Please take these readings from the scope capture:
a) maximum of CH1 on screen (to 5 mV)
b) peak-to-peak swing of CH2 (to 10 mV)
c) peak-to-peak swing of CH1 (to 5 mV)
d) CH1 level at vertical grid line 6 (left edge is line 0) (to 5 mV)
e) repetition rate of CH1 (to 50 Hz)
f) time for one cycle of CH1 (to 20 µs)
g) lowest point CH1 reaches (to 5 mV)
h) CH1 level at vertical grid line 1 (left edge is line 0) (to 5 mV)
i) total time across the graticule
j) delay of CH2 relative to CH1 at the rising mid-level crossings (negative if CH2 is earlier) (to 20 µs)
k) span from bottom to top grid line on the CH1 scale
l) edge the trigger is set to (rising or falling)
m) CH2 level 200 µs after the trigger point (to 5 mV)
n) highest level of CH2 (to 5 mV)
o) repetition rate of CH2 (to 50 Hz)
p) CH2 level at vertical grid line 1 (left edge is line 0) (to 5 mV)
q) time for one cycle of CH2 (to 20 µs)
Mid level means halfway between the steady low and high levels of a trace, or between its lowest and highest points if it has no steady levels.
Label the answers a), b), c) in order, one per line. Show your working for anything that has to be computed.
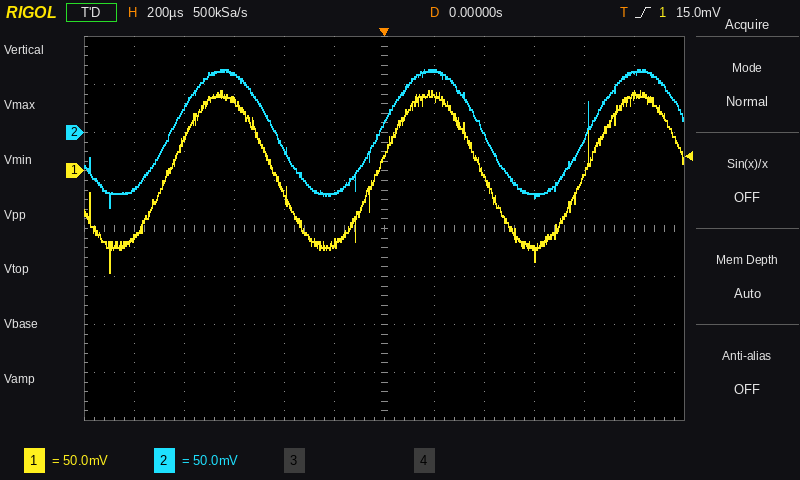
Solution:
a) 85 mV
b) 140 mV
c) 85 mV − (-105 mV) = 190 mV
d) 15 mV
e) 1 / 840 µs ≈ 1.19 kHz, so 1.20 kHz to the nearest 50 Hz
f) 840 µs
g) -105 mV
h) -70 mV
i) 2.4 ms
j) +20 µs
k) 400 mV
l) rising
m) 65 mV
n) 65 mV
o) 1 / 840 µs ≈ 1.19 kHz, so 1.20 kHz to the nearest 50 Hz
p) -60 mV
q) 840 µs
